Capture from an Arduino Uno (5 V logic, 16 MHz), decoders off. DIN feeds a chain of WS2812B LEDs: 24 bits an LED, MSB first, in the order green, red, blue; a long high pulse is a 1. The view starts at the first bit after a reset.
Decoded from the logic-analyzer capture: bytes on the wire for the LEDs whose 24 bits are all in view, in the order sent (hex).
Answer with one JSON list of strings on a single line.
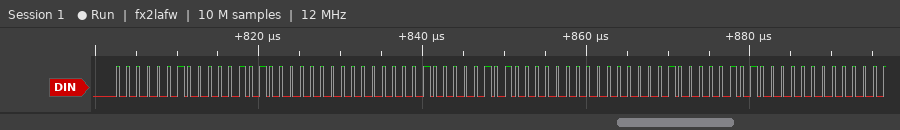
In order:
["02 0A 00 02 0A 00 02 0A 00"]
